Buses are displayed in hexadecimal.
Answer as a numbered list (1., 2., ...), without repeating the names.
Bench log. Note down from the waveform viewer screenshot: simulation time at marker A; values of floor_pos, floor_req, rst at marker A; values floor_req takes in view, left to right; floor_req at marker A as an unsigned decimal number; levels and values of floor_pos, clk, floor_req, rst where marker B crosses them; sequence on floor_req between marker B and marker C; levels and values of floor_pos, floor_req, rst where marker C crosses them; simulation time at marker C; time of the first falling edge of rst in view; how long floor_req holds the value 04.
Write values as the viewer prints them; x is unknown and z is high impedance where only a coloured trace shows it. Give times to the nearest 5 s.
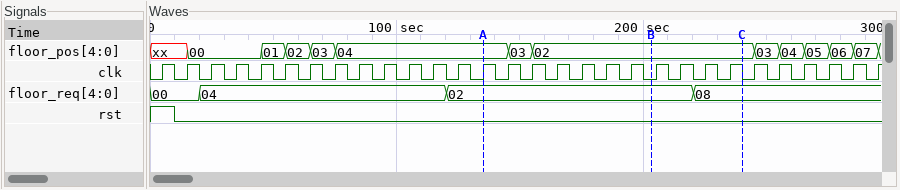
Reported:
1. 135 s
2. floor_pos=04, floor_req=02, rst=0
3. 00, 04, 02, 08
4. 2
5. floor_pos=02, clk=0, floor_req=02, rst=0
6. 02, 08
7. floor_pos=02, floor_req=08, rst=0
8. 240 s
9. 10 s
10. 100 s
